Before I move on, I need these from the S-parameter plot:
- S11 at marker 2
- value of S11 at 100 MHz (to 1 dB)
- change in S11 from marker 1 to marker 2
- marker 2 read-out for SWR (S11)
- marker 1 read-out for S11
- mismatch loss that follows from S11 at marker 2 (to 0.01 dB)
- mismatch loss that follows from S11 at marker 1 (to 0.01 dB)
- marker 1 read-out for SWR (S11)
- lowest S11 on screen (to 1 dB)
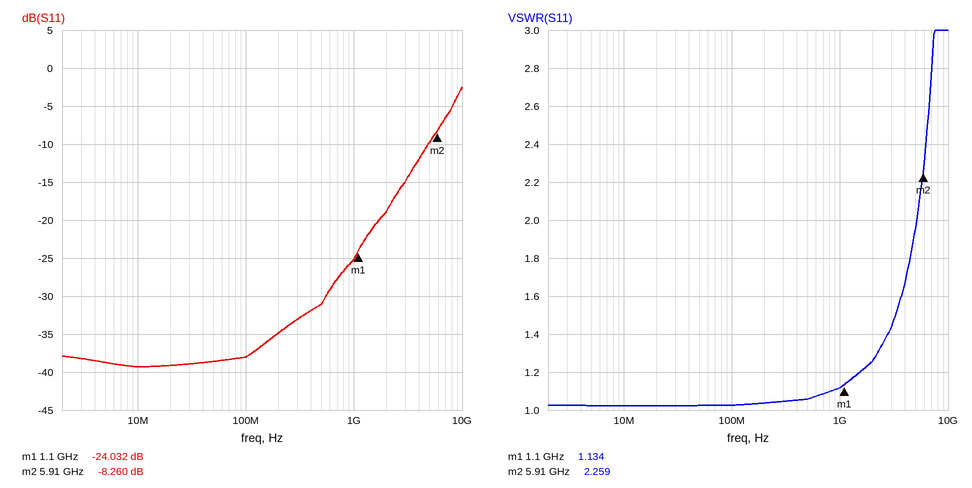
-8.260 dB
-38 dB
15.772 dB
2.259
-24.032 dB
0.70 dB
0.02 dB
1.134
-39 dB
